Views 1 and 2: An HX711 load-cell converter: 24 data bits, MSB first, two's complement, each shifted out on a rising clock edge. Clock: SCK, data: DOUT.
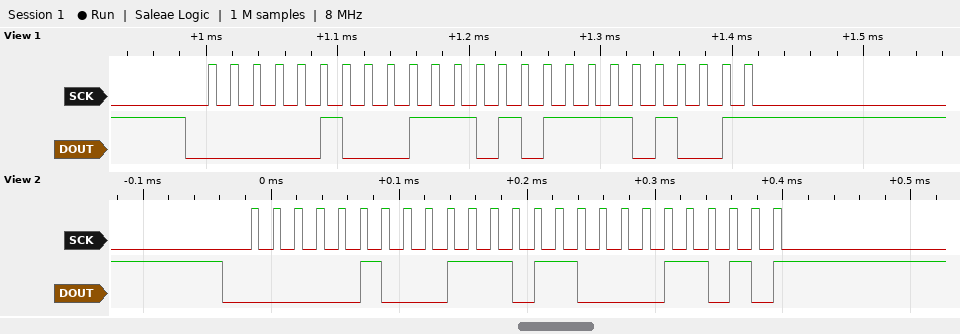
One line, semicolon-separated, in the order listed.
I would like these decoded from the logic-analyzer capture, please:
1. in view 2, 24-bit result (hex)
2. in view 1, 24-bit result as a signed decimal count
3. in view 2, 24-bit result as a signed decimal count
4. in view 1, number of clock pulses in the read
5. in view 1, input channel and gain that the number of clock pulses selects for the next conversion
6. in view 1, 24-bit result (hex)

0x04761A; 292329; 292378; 25; channel A, gain 128; 0x0475E9
